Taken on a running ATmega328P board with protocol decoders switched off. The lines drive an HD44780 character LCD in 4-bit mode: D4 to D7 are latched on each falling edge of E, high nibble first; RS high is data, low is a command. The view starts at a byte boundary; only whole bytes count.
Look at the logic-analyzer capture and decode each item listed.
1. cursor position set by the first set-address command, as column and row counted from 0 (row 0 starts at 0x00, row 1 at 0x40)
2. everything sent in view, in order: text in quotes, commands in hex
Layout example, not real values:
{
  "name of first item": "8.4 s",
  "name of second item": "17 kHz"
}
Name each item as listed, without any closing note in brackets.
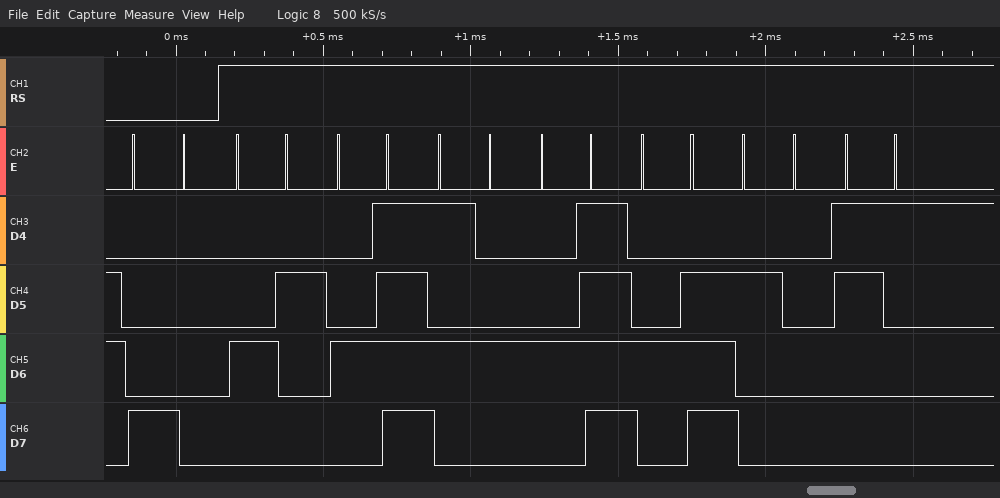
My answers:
{
  "cursor position set by the first set-address command, as column and row counted from 0": "column 0, row 0",
  "everything sent in view, in order: text in quotes, commands in hex": "0x80 \"BOTON 1\""
}
